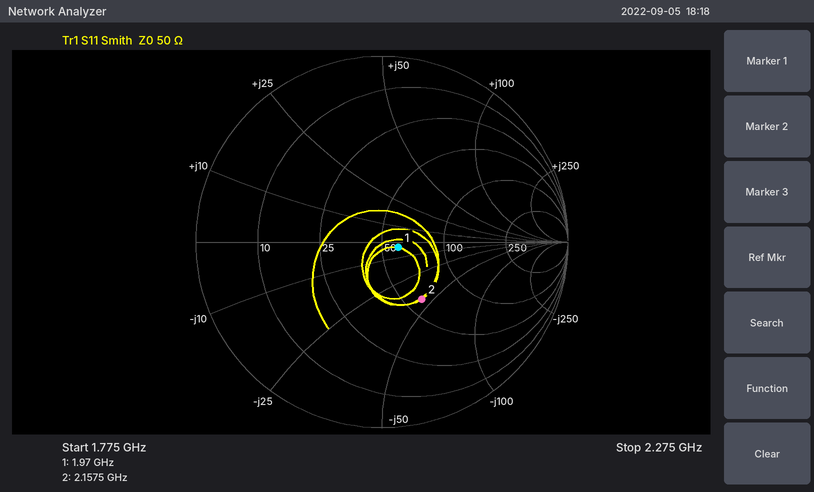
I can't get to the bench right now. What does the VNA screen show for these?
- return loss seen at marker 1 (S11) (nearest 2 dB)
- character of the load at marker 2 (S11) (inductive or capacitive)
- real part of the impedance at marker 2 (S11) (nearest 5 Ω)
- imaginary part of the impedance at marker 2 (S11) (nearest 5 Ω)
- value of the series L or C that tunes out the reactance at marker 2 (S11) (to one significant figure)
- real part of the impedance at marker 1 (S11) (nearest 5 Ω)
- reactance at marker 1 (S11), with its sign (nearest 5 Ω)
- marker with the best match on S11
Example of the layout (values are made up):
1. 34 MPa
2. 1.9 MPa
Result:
1. 20 dB
2. capacitive
3. 60 Ω
4. -45 Ω
5. 3 nH
6. 60 Ω
7. -5 Ω
8. marker 1
